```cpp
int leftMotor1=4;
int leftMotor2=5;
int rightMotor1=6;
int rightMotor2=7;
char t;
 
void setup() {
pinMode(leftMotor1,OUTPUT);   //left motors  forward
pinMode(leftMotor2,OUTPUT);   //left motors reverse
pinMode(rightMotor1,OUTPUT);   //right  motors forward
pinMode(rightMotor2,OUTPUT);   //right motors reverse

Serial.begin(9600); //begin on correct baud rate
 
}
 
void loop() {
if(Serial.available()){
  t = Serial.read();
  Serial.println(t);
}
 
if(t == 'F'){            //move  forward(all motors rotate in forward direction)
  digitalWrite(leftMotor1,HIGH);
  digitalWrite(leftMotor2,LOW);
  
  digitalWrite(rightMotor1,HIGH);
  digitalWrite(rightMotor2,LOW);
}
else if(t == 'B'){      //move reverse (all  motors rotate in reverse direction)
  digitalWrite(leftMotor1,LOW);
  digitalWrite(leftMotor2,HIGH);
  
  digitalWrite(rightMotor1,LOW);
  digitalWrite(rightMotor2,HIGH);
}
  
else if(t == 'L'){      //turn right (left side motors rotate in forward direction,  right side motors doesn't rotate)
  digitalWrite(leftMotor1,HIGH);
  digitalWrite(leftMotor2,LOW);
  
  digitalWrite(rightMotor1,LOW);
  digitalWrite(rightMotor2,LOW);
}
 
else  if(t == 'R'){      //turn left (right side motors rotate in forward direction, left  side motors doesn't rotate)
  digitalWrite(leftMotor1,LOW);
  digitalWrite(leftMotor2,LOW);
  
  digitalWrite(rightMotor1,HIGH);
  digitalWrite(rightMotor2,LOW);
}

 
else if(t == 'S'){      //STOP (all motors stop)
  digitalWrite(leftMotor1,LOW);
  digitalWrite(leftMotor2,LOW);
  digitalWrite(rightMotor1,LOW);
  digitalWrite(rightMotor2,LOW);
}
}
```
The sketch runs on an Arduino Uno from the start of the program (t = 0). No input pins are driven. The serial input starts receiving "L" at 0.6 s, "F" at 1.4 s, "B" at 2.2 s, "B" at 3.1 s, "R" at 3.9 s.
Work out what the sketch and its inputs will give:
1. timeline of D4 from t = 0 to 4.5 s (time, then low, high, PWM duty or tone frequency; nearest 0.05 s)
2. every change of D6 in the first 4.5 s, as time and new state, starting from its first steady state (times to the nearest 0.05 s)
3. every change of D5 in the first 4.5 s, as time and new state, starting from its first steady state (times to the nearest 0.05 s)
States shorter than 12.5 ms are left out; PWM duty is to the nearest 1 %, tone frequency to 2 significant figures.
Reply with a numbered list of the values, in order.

1. 0 s low; 0.6 s high; 2.2 s low
2. 0 s low; 1.4 s high; 2.2 s low; 3.9 s high
3. 0 s low; 2.2 s high; 3.9 s low
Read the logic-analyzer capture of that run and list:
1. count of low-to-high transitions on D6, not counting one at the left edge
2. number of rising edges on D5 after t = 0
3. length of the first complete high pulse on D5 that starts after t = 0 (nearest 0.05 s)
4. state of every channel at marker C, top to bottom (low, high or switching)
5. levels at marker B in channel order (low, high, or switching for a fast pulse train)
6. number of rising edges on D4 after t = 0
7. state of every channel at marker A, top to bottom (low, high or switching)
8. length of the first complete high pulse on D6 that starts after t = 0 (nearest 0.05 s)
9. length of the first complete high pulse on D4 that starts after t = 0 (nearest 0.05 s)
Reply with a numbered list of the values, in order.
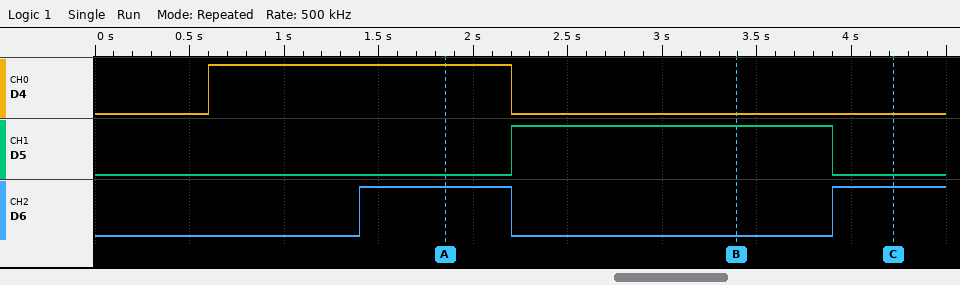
1. 2
2. 1
3. 1.70 s
4. D4 low, D5 low, D6 high
5. D4 low, D5 high, D6 low
6. 1
7. D4 high, D5 low, D6 high
8. 0.80 s
9. 1.60 s
